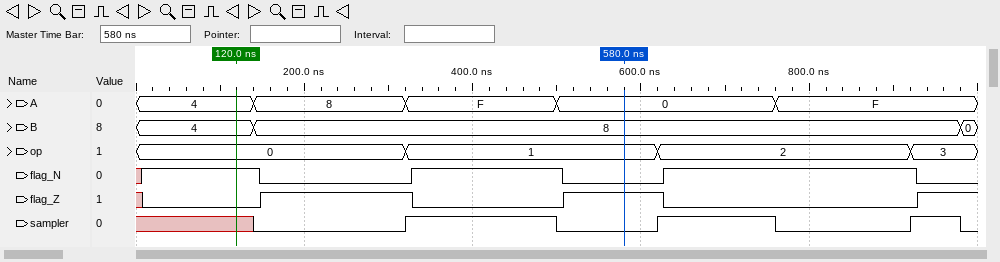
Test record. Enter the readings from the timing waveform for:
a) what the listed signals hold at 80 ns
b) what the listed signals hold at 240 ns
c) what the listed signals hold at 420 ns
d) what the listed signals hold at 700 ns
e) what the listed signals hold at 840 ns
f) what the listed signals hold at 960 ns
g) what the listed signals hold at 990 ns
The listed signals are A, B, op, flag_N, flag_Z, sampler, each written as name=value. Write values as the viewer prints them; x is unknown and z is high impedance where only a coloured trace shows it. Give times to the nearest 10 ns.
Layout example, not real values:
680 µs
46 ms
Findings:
A=4, B=4, op=0, flag_N=1, flag_Z=0, sampler=x
A=8, B=8, op=0, flag_N=0, flag_Z=1, sampler=0
A=F, B=8, op=1, flag_N=1, flag_Z=0, sampler=1
A=0, B=8, op=2, flag_N=1, flag_Z=0, sampler=1
A=F, B=8, op=2, flag_N=1, flag_Z=0, sampler=0
A=F, B=8, op=3, flag_N=0, flag_Z=1, sampler=1
A=F, B=0, op=3, flag_N=0, flag_Z=1, sampler=0
